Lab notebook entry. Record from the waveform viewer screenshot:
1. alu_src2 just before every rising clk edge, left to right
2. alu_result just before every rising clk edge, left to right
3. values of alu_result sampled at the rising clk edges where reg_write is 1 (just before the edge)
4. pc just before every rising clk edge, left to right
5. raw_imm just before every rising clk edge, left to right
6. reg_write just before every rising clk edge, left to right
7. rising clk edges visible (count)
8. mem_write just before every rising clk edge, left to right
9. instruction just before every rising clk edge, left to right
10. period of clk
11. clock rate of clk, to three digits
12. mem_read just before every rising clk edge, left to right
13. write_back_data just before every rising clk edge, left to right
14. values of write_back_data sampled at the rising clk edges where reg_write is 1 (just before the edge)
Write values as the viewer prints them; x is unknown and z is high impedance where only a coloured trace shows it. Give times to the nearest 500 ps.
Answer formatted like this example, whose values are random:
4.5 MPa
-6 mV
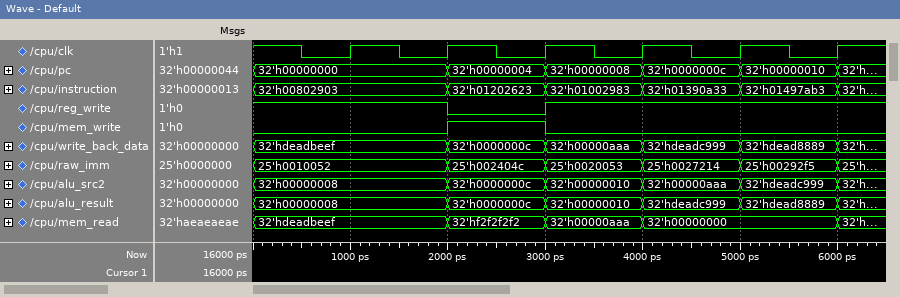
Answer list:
32'h00000008, 32'h00000008, 32'h0000000c, 32'h00000010, 32'h00000aaa, 32'hdeadc999
32'h00000008, 32'h00000008, 32'h0000000c, 32'h00000010, 32'hdeadc999, 32'hdead8889
32'h00000008, 32'h00000008, 32'h00000010, 32'hdeadc999, 32'hdead8889
32'h00000000, 32'h00000000, 32'h00000004, 32'h00000008, 32'h0000000c, 32'h00000010
25'h0010052, 25'h0010052, 25'h002404c, 25'h0020053, 25'h0027214, 25'h00292f5
1 1 0 1 1 1
6
0 0 1 0 0 0
32'h00802903, 32'h00802903, 32'h01202623, 32'h01002983, 32'h01390a33, 32'h01497ab3
1000 ps
1.00 GHz
32'hdeadbeef, 32'hdeadbeef, 32'hf2f2f2f2, 32'h00000aaa, 32'h00000000, 32'h00000000
32'hdeadbeef, 32'hdeadbeef, 32'h0000000c, 32'h00000aaa, 32'hdeadc999, 32'hdead8889
32'hdeadbeef, 32'hdeadbeef, 32'h00000aaa, 32'hdeadc999, 32'hdead8889
